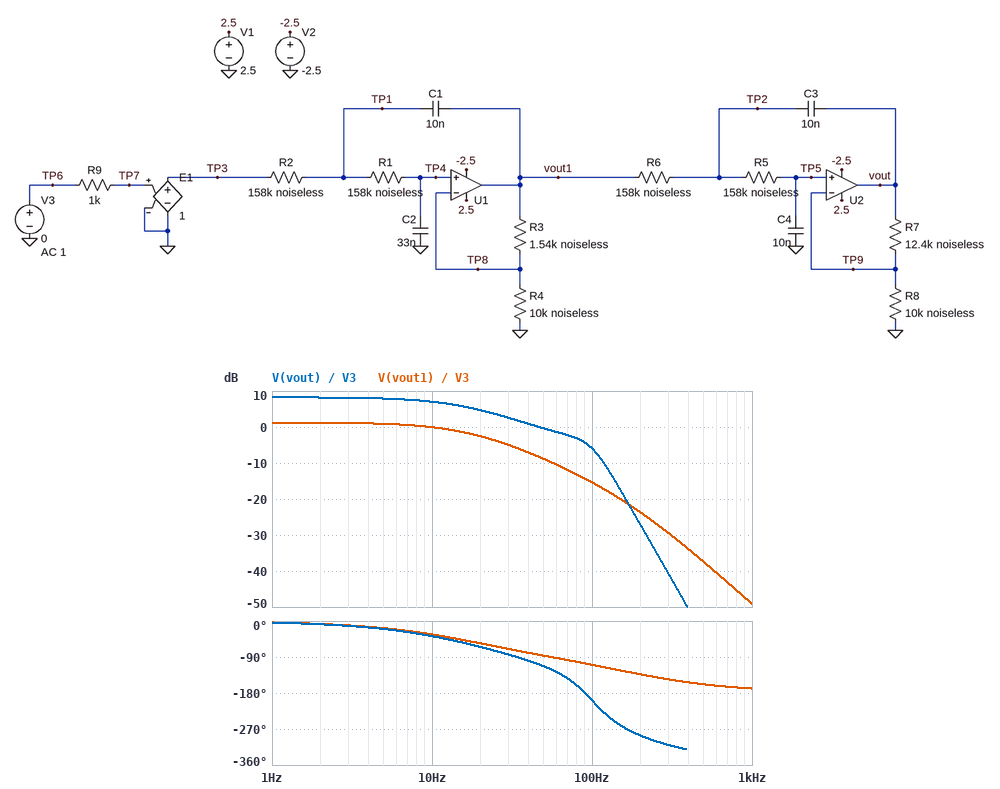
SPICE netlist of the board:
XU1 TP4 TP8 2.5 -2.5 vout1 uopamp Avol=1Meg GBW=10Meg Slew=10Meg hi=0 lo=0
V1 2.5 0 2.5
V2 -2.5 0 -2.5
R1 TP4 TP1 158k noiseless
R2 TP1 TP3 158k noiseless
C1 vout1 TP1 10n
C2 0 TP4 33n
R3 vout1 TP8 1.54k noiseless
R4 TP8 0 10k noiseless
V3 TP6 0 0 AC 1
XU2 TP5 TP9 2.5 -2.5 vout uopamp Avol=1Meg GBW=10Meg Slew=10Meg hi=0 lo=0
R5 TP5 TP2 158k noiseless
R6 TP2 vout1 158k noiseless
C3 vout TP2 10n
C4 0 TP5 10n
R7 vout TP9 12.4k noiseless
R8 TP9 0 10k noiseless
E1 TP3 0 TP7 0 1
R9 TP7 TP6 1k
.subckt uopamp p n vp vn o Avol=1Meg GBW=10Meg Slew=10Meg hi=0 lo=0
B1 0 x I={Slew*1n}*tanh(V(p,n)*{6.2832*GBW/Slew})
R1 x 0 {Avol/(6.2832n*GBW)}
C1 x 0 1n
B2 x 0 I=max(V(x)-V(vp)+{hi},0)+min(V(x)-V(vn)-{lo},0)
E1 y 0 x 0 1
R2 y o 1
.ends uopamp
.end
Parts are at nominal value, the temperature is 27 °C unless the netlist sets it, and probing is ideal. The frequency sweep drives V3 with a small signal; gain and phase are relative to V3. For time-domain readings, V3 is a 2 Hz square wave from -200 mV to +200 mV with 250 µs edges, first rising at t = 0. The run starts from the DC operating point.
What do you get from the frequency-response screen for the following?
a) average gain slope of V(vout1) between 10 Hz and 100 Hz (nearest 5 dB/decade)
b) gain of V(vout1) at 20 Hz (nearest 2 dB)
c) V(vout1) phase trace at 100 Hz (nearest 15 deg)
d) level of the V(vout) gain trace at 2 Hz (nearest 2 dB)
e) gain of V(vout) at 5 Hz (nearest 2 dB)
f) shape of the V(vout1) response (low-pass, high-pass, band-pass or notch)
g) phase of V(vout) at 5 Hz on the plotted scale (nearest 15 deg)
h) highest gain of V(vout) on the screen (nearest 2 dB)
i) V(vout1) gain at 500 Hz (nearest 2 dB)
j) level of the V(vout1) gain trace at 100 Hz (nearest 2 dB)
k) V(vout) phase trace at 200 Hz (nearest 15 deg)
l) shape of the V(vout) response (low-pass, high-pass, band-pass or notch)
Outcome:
-15 dB/decade
-2 dB
-105 deg
8 dB
8 dB
low-pass
-15 deg
8 dB
-38 dB
-16 dB
-285 deg
low-pass
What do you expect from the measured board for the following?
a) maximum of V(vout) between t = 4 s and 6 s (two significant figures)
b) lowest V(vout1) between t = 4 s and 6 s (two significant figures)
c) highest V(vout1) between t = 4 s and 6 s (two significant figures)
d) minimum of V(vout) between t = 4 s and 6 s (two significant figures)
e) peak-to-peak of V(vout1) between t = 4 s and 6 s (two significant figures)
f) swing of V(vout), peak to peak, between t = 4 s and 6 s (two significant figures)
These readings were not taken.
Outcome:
520 mV
-230 mV
230 mV
-520 mV
460 mV
1.0 V
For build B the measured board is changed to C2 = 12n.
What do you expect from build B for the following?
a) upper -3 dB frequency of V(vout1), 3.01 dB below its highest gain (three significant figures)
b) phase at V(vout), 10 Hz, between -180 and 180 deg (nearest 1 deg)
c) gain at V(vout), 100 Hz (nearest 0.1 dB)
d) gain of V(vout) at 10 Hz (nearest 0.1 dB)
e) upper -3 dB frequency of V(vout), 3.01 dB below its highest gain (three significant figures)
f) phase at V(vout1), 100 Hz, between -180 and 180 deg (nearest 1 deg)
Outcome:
57.1 Hz
-17 deg
3.7 dB
8.2 dB
89.6 Hz
-95 deg
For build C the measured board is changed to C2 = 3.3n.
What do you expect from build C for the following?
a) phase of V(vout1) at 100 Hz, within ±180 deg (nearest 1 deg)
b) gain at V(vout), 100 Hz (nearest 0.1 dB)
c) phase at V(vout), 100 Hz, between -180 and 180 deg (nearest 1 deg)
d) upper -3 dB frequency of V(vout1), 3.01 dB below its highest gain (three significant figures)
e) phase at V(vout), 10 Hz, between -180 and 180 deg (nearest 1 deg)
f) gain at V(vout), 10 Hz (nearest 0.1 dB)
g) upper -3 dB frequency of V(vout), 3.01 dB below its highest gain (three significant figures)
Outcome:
-37 deg
12.2 dB
-126 deg
208 Hz
-7 deg
8.3 dB
125 Hz
